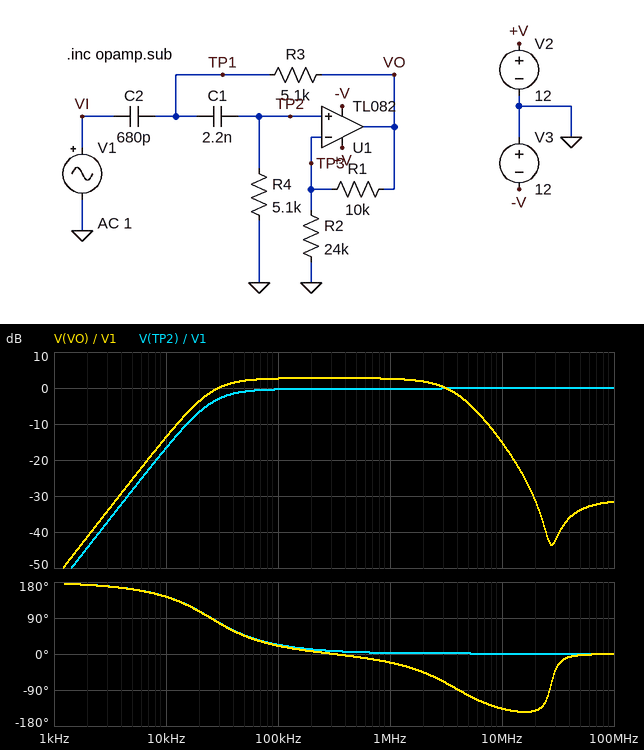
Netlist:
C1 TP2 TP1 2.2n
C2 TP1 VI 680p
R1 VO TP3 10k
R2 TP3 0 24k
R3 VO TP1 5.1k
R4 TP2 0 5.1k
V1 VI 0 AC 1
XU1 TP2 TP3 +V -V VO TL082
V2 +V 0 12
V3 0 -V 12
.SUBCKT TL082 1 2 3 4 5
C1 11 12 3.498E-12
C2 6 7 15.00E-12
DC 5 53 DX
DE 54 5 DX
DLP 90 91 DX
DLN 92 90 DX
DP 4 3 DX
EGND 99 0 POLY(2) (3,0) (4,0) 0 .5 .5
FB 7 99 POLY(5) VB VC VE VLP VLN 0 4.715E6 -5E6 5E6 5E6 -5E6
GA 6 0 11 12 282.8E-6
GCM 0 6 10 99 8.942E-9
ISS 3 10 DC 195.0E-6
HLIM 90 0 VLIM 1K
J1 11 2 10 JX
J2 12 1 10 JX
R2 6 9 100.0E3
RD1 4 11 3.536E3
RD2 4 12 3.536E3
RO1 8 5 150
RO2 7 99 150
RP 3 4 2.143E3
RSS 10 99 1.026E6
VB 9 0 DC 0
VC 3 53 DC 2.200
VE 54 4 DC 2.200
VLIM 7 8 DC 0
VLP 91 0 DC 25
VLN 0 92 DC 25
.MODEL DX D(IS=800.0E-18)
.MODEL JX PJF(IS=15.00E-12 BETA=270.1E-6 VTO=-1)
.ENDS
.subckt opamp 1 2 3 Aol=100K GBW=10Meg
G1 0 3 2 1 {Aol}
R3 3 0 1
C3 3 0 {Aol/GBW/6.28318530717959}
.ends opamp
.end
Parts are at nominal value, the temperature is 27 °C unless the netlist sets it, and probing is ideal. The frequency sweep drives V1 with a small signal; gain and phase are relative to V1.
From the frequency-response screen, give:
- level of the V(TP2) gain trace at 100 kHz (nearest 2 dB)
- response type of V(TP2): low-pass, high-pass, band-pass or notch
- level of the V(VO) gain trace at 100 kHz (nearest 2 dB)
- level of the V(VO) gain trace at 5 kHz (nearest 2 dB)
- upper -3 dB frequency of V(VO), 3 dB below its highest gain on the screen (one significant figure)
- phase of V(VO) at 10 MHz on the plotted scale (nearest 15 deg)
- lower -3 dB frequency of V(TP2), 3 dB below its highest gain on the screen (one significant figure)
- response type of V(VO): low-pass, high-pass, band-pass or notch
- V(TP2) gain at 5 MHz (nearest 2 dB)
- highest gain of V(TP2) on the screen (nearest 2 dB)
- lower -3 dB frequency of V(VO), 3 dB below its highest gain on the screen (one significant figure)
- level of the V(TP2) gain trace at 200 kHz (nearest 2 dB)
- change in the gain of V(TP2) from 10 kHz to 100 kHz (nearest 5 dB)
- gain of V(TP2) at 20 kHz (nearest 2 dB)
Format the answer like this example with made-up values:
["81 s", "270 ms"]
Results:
["0 dB", "high-pass", "2 dB", "-26 dB", "3 MHz", "-135 deg", "30 kHz", "band-pass", "0 dB", "0 dB", "30 kHz", "0 dB", "15 dB", "-6 dB"]
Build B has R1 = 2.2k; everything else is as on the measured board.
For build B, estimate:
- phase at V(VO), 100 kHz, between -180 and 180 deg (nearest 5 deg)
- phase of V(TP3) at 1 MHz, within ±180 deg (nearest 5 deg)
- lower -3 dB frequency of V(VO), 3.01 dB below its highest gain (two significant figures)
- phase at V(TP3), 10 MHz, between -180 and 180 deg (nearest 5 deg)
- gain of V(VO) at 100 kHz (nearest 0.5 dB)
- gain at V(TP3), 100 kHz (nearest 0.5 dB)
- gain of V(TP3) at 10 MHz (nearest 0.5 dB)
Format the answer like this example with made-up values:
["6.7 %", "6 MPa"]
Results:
["30 deg", "-15 deg", "44 kHz", "-135 deg", "0 dB", "-1.0 dB", "-15.5 dB"]
